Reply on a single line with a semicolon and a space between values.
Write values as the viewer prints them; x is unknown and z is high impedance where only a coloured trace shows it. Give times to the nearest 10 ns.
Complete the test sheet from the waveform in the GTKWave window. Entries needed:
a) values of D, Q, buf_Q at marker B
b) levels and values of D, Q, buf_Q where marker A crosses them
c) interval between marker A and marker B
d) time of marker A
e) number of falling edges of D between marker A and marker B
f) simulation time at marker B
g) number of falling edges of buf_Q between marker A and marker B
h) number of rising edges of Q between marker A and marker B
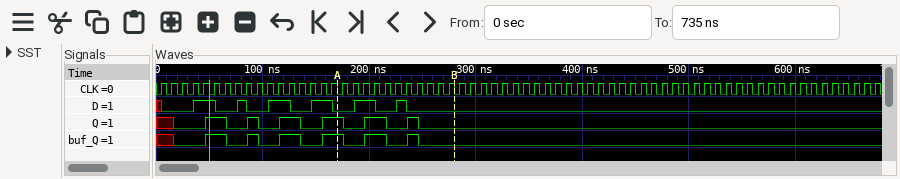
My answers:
D=0, Q=0, buf_Q=0; D=0, Q=1, buf_Q=1; 110 ns; 170 ns; 2; 280 ns; 3; 2
